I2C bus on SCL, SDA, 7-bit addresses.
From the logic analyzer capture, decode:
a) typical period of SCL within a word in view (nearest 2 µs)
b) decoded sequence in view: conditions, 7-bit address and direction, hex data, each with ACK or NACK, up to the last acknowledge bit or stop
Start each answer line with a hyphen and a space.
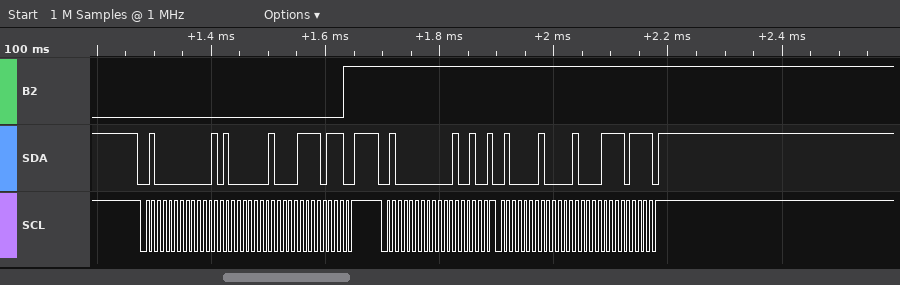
- 10 µs
- start, address 20 write ACK, 14 ACK, 08 ACK, F7 ACK, stop, start, address 20 write ACK, 12 ACK, repeated start, address 20 read ACK, 08 ACK, F7 NACK, stop
